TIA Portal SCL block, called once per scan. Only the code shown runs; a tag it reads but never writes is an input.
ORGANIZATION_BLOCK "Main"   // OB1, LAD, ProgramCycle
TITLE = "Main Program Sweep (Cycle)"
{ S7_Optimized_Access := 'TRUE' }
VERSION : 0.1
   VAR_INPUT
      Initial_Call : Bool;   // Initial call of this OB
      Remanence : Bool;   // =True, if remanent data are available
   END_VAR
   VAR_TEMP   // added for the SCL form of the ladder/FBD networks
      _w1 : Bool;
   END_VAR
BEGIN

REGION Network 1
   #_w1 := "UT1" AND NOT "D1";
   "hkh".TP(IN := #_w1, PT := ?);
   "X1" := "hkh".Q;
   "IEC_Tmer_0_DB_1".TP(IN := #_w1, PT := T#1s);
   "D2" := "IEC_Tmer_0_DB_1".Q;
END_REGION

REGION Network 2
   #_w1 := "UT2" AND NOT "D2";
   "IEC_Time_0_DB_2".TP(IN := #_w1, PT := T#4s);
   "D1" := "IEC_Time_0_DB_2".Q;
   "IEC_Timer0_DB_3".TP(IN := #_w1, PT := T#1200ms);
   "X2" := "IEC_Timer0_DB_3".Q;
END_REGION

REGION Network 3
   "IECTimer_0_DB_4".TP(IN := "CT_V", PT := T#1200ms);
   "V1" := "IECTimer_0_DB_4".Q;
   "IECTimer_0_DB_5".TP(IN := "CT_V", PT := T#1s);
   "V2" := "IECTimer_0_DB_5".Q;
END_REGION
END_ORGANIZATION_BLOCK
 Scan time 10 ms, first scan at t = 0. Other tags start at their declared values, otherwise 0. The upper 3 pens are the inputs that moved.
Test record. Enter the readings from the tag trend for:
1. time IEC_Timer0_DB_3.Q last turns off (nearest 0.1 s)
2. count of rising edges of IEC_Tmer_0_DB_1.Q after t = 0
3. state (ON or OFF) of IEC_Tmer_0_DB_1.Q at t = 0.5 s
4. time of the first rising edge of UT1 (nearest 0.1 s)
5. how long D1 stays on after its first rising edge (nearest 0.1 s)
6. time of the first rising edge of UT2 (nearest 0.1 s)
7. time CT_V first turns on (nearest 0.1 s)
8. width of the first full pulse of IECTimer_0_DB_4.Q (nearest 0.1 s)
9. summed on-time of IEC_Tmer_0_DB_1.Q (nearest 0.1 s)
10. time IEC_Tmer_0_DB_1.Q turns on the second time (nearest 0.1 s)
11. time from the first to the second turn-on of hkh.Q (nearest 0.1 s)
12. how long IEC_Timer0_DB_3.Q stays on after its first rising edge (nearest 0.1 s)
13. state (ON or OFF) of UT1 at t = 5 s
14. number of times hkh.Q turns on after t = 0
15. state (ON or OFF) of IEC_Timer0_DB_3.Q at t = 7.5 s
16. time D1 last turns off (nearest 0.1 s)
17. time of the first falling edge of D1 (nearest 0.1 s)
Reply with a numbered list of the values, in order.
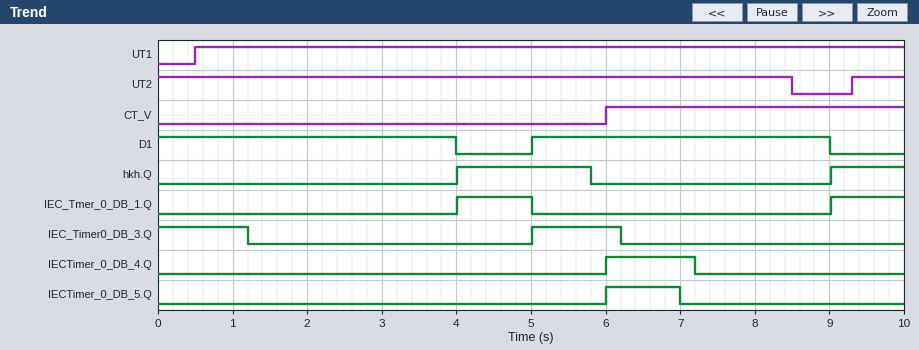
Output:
1. 6.2 s
2. 2
3. OFF
4. 0.5 s
5. 4.0 s
6. 9.3 s
7. 6.0 s
8. 1.2 s
9. 2.0 s
10. 9.0 s
11. 5.0 s
12. 1.2 s
13. ON
14. 2
15. OFF
16. 9.0 s
17. 4.0 s
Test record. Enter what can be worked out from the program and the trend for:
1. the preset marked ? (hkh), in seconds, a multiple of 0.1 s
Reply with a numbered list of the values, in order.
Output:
1. 1.8 s
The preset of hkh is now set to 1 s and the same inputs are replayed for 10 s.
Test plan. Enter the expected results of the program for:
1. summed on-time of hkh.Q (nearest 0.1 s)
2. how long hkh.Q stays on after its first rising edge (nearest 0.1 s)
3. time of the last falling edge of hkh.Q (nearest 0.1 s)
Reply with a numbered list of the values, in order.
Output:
1. 2.0 s
2. 1.0 s
3. 5.0 s
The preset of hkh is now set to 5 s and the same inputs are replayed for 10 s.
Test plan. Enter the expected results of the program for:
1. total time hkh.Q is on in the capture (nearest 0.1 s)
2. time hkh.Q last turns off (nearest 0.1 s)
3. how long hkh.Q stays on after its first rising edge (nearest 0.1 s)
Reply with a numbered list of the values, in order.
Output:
1. 6.0 s
2. 9.0 s
3. 5.0 s
